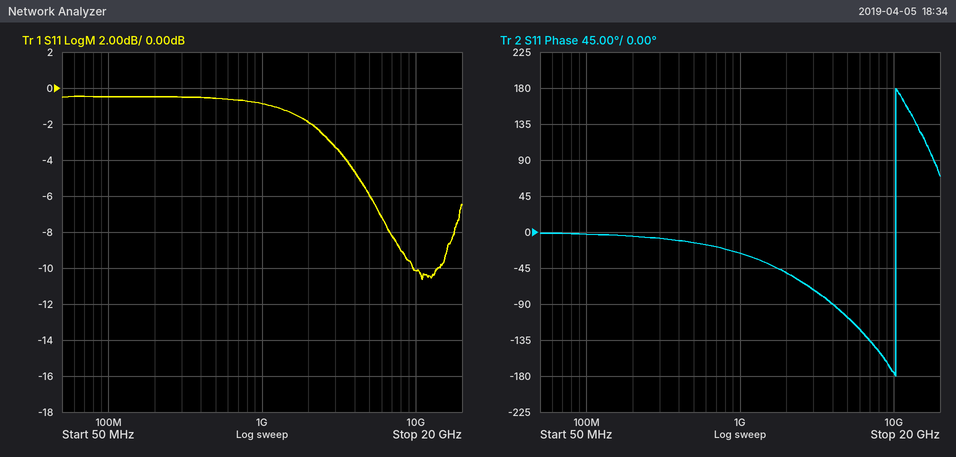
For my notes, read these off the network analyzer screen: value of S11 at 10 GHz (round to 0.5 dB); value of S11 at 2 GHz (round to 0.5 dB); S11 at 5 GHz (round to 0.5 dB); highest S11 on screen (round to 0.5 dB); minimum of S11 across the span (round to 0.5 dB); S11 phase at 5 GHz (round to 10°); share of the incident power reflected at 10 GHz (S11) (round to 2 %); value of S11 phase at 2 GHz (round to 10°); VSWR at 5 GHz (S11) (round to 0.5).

-10.0 dB
-2.0 dB
-6.0 dB
-0.5 dB
-10.5 dB
-110°
10 %
-50°
3.0
